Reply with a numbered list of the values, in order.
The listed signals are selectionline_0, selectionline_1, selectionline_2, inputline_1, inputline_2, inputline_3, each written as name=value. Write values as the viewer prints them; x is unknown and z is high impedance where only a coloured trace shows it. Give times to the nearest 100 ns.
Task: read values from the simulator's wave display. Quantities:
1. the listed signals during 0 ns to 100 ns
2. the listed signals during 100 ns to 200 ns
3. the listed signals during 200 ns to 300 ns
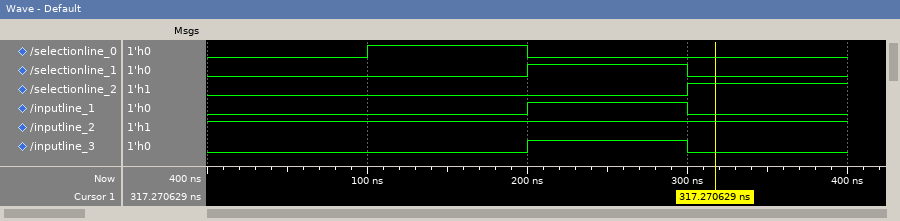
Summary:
1. selectionline_0=0, selectionline_1=0, selectionline_2=0, inputline_1=0, inputline_2=1, inputline_3=0
2. selectionline_0=1, selectionline_1=0, selectionline_2=0, inputline_1=0, inputline_2=1, inputline_3=0
3. selectionline_0=0, selectionline_1=1, selectionline_2=0, inputline_1=1, inputline_2=1, inputline_3=1
